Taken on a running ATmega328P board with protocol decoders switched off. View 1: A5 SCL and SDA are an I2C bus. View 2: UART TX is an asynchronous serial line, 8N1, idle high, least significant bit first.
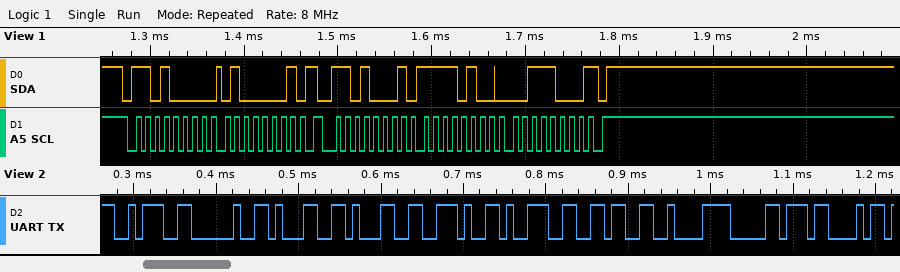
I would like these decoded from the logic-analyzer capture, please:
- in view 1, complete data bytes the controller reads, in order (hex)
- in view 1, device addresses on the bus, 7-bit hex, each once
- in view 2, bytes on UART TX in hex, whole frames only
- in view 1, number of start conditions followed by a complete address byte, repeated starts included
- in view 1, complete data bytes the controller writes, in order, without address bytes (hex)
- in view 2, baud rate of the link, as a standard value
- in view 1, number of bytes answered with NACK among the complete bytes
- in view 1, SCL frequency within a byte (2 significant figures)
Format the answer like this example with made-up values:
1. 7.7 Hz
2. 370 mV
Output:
1. F4 38
2. 0x68
3. 3A 20 31 31 2E 39 36 C2 B0 43
4. 2
5. 41
6. 115200 baud
7. 1
8. 100 kHz
